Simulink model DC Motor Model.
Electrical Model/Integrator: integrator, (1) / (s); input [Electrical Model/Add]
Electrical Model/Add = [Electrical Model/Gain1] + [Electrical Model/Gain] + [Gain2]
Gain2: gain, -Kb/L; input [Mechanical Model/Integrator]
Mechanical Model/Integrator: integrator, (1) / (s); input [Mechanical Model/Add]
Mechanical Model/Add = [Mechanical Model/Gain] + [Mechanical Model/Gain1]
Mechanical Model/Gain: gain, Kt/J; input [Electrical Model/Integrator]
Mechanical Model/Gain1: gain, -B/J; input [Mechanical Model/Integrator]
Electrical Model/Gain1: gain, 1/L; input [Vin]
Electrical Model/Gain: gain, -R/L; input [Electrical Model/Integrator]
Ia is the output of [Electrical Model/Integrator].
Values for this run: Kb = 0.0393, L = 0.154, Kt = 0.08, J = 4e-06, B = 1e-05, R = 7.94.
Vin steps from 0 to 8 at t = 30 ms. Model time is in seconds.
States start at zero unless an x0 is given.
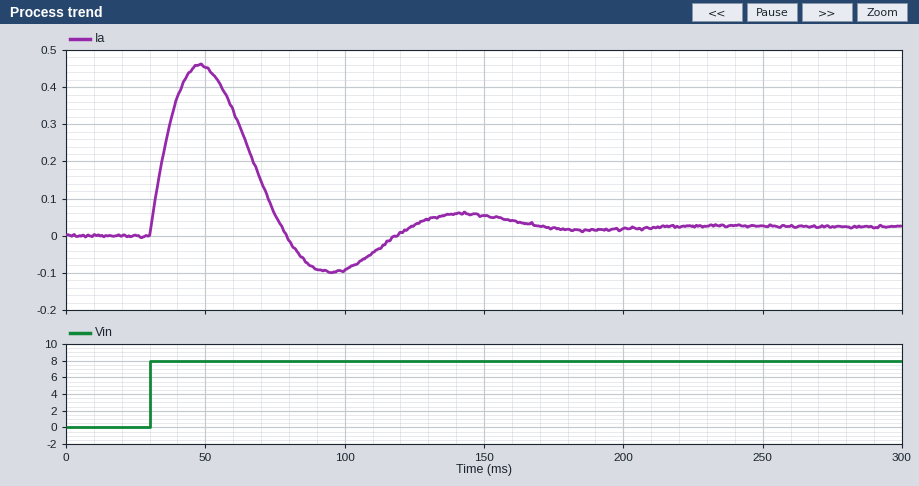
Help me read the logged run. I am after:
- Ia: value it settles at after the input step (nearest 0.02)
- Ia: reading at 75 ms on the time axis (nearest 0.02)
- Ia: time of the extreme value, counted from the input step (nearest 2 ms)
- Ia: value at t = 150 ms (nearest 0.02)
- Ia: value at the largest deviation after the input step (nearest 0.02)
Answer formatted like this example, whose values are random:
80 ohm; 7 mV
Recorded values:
0.02; 0.06; 18 ms; 0.06; 0.46
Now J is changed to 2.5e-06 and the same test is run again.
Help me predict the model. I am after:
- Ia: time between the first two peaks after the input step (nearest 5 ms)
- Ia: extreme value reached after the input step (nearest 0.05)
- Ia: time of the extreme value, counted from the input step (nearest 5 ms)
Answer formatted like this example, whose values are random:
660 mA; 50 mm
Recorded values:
70 ms; 0.40; 15 ms
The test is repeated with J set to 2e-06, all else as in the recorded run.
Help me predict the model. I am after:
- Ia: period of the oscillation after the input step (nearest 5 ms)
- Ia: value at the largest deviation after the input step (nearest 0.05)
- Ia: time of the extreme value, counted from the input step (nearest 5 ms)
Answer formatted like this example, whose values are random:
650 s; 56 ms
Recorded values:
65 ms; 0.35; 15 ms
